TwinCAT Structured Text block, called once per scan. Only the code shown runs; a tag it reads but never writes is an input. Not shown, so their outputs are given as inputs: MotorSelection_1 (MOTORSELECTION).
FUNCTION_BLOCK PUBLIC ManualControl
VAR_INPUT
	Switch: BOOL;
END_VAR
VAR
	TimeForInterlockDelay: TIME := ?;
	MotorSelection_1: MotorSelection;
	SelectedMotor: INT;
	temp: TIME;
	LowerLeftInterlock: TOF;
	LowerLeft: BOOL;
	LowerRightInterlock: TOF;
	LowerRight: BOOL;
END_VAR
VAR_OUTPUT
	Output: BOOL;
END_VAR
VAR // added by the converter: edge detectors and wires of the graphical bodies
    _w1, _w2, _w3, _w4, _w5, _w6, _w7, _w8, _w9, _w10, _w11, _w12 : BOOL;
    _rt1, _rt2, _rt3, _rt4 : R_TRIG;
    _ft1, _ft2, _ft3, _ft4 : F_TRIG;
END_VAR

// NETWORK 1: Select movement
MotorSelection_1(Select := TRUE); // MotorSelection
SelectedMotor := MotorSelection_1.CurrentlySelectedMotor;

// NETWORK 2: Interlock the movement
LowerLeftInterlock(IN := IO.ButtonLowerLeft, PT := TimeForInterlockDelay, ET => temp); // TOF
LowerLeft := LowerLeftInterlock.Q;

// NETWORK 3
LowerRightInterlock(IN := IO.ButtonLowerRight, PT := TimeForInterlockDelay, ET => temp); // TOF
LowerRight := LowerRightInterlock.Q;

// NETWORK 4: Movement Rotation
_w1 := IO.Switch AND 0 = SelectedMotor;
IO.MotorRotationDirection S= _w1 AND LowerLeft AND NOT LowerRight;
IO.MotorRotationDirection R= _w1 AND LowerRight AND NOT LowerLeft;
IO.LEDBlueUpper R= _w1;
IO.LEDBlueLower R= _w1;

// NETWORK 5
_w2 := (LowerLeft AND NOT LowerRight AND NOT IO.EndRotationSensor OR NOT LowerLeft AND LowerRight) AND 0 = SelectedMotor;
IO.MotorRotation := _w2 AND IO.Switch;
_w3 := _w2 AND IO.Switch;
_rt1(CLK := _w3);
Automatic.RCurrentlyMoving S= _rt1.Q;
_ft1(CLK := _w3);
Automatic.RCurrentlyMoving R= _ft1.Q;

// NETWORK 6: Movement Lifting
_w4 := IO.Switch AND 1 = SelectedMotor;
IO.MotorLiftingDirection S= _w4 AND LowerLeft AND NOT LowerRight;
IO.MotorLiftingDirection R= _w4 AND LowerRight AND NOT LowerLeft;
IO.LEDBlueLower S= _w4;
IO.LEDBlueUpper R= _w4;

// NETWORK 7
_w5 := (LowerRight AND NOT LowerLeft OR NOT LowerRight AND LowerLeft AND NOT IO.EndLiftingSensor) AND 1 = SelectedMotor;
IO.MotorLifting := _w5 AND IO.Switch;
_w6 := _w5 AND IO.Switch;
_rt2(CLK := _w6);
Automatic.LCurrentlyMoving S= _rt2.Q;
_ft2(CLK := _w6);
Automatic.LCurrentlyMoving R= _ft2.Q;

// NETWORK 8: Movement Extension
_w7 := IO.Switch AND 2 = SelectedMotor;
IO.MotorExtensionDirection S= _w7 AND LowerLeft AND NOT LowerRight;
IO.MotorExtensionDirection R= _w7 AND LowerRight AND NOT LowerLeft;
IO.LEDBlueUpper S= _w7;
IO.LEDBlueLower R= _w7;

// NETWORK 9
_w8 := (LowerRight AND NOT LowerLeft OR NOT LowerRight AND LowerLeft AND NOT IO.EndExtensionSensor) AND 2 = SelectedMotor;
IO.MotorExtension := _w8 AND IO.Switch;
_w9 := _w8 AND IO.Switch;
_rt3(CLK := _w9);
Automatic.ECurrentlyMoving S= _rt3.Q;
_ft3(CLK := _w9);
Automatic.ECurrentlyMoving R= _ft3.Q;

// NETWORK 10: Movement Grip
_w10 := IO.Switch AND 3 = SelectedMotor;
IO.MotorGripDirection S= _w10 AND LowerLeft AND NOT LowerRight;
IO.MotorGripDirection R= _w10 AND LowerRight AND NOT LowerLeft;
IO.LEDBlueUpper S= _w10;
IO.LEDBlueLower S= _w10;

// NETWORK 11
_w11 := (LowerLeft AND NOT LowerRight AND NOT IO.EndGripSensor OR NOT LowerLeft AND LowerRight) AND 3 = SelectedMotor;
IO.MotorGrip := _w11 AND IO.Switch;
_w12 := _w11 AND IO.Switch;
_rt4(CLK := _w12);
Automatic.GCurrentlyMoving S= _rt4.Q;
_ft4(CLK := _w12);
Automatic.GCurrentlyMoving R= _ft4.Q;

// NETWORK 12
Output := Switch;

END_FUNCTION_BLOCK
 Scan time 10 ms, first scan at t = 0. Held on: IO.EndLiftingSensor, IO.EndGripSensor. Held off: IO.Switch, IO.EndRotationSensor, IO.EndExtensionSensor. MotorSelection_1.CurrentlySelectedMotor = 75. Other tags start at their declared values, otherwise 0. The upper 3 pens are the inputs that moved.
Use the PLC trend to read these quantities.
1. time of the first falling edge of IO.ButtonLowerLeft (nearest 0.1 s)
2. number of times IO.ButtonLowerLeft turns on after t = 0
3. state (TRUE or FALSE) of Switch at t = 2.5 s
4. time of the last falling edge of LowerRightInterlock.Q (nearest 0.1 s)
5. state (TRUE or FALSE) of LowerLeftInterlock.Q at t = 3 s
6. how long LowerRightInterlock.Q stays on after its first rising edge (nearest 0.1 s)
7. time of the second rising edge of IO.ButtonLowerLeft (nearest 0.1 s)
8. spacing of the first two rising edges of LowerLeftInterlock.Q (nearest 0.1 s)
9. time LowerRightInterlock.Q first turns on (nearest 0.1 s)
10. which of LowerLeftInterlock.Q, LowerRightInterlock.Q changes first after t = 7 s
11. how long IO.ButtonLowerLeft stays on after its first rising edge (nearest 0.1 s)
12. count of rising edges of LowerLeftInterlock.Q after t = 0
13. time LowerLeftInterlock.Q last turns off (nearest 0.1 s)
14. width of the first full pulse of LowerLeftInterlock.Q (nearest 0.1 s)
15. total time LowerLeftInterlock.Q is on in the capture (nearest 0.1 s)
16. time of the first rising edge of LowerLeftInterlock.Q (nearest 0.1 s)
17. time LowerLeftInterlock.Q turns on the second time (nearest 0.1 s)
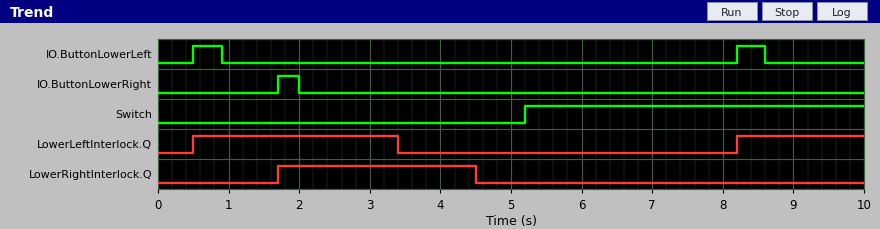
0.9 s
2
FALSE
4.5 s
TRUE
2.8 s
8.2 s
7.7 s
1.7 s
LowerLeftInterlock.Q
0.4 s
2
3.4 s
2.9 s
4.7 s
0.5 s
8.2 s
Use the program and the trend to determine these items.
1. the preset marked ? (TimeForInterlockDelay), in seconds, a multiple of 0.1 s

2.5 s
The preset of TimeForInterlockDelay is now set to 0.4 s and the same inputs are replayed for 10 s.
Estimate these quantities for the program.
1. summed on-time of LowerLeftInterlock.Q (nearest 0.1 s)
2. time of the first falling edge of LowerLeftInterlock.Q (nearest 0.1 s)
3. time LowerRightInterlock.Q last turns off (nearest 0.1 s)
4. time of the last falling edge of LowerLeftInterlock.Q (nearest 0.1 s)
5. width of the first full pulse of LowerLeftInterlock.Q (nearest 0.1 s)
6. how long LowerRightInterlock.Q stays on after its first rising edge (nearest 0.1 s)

1.6 s
1.3 s
2.4 s
9.0 s
0.8 s
0.7 s
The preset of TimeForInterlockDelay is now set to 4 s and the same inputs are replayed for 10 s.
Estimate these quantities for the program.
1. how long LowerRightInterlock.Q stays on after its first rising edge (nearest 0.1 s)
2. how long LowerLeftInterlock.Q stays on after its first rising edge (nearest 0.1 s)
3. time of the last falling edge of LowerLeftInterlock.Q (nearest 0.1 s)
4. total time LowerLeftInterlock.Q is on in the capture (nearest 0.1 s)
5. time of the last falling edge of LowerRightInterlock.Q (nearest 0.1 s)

4.3 s
4.4 s
4.9 s
6.2 s
6.0 s
